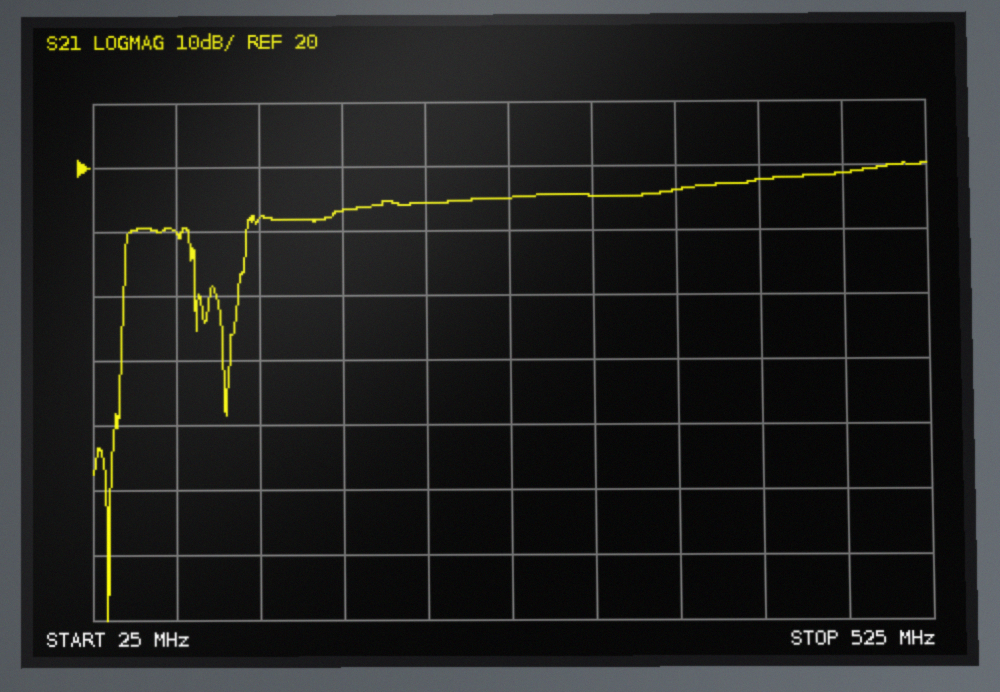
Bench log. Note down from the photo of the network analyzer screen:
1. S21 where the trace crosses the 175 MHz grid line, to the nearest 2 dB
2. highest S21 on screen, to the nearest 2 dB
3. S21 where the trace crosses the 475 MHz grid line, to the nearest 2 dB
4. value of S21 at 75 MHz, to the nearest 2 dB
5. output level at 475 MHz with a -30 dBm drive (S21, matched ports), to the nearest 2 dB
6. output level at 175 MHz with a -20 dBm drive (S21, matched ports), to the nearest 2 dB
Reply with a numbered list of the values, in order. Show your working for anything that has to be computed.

1. 14 dB
2. 20 dB
3. 18 dB
4. 10 dB
5. -30 dBm + (18 dB) = -12 dBm
6. -20 dBm + (14 dB) = -6 dBm
